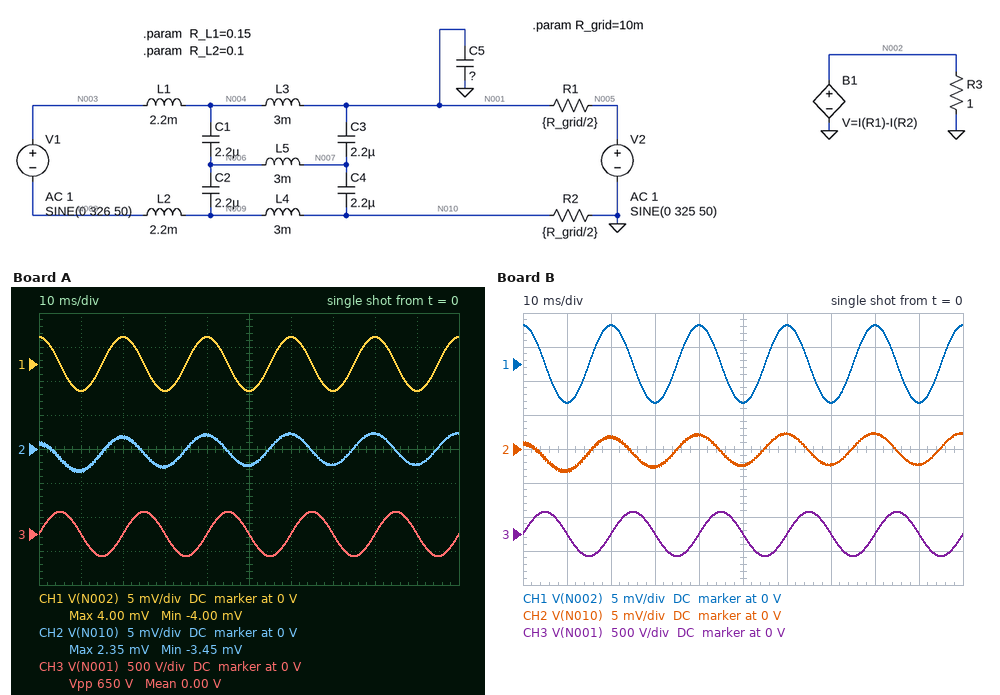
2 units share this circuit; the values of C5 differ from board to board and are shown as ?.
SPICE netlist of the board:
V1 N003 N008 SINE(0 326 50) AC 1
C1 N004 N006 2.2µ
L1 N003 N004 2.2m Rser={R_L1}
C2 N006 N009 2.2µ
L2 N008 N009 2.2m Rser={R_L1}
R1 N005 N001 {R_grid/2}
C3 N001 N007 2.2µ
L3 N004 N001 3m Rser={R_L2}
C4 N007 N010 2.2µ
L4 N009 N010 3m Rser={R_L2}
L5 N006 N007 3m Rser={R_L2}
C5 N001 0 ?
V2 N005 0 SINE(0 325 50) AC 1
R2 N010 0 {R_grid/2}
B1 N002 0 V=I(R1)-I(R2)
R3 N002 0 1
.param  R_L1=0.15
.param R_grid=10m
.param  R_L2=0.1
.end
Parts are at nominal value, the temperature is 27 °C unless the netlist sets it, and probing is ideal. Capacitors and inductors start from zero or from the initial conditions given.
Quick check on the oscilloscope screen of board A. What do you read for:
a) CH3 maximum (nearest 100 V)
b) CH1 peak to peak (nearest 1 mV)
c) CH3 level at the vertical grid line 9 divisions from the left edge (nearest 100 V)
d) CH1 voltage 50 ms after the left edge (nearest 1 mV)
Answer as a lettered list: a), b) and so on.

a) 300 V
b) 8 mV
c) 0 V
d) -4 mV
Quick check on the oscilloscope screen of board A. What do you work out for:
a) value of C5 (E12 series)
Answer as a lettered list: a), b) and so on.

a) 39 nF
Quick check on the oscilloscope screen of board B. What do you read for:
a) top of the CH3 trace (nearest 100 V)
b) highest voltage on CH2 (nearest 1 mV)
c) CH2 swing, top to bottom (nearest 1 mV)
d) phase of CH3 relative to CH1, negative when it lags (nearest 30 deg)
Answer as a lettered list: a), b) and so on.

a) 300 V
b) 2 mV
c) 6 mV
d) -90 deg
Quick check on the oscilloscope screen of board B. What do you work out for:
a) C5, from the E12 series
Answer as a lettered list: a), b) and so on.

a) 56 nF
